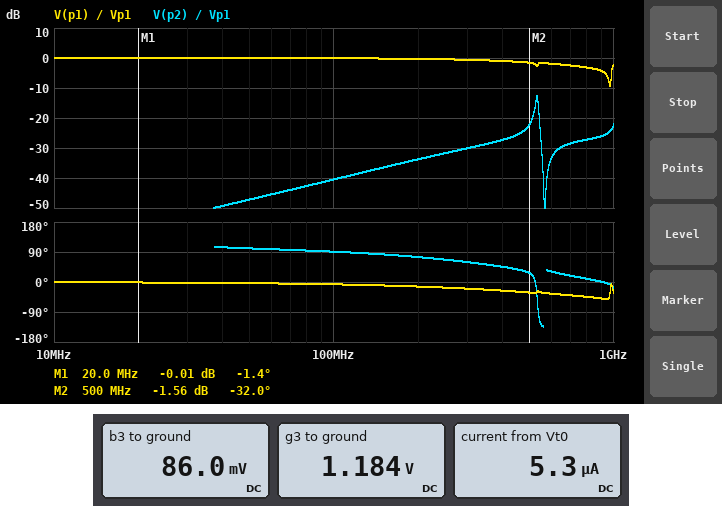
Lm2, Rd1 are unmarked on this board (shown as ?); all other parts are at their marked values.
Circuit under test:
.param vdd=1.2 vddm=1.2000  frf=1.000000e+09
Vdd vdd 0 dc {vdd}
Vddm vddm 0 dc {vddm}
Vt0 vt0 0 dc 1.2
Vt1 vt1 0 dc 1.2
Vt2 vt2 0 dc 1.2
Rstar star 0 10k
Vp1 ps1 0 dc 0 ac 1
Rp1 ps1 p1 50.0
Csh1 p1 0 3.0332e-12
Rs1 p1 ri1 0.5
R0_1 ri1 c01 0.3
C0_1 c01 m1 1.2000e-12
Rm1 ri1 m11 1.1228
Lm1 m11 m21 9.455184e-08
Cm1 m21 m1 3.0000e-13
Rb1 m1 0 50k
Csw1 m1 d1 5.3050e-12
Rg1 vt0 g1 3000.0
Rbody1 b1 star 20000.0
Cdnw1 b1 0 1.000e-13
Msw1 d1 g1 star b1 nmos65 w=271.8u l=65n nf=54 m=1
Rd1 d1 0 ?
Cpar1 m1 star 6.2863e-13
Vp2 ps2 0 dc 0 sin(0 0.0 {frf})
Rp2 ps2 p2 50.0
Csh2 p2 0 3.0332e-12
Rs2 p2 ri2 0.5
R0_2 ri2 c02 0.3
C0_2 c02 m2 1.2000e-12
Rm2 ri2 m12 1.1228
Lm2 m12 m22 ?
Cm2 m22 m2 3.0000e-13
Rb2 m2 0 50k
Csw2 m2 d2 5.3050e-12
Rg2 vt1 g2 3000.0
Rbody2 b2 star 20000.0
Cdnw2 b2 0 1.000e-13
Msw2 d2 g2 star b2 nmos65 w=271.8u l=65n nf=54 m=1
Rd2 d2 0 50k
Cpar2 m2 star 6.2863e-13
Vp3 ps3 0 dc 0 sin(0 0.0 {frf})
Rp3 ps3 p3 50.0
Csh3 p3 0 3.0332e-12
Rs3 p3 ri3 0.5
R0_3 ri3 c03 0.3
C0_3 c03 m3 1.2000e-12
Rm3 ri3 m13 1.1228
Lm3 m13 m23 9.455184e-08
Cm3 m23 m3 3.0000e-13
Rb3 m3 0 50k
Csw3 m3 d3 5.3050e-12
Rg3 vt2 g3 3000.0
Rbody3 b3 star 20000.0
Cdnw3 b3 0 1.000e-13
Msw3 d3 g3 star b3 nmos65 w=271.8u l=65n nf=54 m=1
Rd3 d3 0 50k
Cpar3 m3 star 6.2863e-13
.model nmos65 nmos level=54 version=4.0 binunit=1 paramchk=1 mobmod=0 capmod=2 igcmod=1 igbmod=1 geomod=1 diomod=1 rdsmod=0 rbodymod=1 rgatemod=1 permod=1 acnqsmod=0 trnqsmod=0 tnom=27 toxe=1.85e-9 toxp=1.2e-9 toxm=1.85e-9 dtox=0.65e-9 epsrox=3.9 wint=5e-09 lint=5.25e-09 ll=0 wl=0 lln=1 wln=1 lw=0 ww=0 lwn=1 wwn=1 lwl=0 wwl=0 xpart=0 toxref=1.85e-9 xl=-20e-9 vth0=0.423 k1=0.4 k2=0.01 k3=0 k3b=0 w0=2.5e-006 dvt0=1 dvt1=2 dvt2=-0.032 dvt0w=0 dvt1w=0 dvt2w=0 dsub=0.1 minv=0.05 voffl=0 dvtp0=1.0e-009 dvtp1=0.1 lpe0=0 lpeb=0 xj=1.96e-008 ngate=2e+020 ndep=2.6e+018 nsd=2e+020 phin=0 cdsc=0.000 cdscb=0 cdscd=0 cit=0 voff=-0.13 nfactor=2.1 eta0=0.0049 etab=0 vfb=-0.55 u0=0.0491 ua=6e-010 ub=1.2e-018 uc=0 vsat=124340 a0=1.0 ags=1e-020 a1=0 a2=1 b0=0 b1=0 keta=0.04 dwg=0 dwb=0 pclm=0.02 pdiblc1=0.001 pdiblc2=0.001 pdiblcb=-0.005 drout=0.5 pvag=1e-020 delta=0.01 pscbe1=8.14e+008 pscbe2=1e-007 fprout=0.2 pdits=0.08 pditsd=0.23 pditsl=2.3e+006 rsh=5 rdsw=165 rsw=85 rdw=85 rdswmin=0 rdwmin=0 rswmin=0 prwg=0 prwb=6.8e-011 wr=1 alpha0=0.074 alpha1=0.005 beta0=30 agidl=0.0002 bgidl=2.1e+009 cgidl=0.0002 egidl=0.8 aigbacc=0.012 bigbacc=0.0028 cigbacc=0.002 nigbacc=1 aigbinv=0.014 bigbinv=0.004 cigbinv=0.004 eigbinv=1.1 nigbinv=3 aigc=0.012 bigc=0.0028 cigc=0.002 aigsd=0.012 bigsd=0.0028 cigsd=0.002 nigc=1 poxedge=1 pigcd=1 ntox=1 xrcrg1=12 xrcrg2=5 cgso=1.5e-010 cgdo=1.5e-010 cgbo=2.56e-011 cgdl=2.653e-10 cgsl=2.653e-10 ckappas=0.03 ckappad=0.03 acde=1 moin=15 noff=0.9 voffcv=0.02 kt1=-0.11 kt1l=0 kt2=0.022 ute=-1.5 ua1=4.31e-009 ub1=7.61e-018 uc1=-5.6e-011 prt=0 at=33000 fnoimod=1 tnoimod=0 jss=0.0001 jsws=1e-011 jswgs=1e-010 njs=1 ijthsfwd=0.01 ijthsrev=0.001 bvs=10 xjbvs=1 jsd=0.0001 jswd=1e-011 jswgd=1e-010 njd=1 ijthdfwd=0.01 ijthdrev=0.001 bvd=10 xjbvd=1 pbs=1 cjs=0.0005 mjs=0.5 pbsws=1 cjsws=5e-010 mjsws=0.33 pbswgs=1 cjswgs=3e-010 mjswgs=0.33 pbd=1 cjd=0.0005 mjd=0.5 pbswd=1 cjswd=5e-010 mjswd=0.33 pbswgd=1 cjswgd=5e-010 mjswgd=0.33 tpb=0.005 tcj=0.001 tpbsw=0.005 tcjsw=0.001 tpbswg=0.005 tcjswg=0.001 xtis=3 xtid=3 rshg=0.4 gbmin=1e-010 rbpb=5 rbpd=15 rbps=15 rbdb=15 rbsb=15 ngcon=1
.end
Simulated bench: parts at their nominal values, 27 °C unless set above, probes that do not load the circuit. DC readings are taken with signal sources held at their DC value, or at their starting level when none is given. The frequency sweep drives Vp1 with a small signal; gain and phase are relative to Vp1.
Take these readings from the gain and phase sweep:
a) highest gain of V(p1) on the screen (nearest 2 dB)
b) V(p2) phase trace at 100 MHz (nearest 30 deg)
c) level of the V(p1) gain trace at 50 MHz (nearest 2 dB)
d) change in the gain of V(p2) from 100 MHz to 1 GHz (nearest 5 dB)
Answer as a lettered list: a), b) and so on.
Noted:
a) 0 dB
b) 90 deg
c) 0 dB
d) 20 dB
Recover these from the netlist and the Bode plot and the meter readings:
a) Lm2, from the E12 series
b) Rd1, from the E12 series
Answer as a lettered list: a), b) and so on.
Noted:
a) 330 nH
b) 22 kΩ
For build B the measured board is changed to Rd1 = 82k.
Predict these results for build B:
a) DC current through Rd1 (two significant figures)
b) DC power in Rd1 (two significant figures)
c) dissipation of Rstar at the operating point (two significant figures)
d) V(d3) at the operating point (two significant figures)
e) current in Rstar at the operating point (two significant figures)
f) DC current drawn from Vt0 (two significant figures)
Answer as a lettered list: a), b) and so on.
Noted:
a) 1.2 µA
b) 120 nW
c) 960 nW
d) 98 mV
e) 9.8 µA
f) 5.0 µA
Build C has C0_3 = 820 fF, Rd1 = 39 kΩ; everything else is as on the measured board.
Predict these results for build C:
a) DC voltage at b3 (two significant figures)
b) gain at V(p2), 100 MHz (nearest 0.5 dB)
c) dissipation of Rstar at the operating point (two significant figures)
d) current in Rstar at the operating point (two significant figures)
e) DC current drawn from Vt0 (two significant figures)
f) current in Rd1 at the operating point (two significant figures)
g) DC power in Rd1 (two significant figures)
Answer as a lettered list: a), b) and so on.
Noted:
a) 93 mV
b) -40.0 dB
c) 860 nW
d) 9.3 µA
e) 5.1 µA
f) 2.4 µA
g) 220 nW
